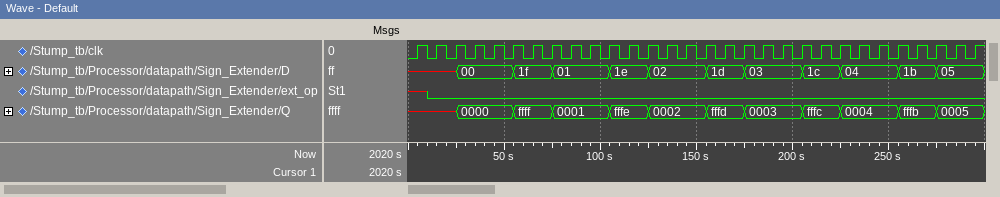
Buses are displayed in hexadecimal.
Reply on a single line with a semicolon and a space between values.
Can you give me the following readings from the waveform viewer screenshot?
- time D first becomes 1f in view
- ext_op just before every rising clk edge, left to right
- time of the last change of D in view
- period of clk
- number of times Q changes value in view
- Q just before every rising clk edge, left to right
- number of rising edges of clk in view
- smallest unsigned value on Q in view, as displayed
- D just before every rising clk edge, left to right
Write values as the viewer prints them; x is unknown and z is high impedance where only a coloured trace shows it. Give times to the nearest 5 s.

55 s; x 0 0 0 0 0 0 0 0 0 0 0 0 0 0 0 0 0 0 0 0 0 0 0 0 0 0 0 0 0; 275 s; 10 s; 11; x, x, x, 0000, 0000, 0000, ffff, ffff, 0001, 0001, 0001, fffe, fffe, 0002, 0002, 0002, fffd, fffd, 0003, 0003, 0003, fffc, fffc, 0004, 0004, 0004, fffb, fffb, 0005, 0005; 30; 0000; x, x, x, 00, 00, 00, 1f, 1f, 01, 01, 01, 1e, 1e, 02, 02, 02, 1d, 1d, 03, 03, 03, 1c, 1c, 04, 04, 04, 1b, 1b, 05, 05
